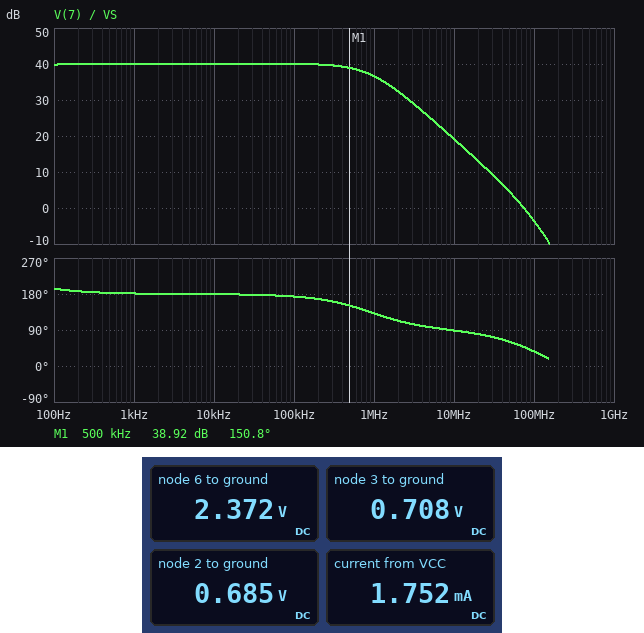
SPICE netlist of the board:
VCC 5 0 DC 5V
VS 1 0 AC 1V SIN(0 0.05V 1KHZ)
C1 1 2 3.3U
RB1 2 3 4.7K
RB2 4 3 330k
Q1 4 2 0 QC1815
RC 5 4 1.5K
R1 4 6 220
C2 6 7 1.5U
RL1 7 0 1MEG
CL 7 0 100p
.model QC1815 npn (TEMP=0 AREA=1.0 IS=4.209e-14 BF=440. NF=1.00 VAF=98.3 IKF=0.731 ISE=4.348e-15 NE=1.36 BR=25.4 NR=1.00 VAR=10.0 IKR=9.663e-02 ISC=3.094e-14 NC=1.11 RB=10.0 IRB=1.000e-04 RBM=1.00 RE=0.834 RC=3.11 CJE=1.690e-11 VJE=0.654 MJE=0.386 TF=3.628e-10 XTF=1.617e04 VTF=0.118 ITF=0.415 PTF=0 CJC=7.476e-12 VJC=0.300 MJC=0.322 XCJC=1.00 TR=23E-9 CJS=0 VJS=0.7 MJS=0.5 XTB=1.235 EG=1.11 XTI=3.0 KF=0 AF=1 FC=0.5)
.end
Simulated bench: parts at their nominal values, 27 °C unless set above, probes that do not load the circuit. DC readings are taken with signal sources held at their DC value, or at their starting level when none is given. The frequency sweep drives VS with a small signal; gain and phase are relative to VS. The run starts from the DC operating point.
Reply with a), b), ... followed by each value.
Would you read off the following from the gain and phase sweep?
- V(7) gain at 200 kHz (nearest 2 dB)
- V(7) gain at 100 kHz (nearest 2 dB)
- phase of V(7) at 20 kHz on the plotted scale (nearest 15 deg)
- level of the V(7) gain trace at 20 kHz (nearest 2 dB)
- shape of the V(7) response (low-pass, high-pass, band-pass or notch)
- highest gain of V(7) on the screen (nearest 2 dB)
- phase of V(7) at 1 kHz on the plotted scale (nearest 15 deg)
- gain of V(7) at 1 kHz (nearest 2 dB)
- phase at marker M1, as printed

a) 40 dB
b) 40 dB
c) 180 deg
d) 40 dB
e) low-pass
f) 40 dB
g) 180 deg
h) 40 dB
i) 150.8 deg
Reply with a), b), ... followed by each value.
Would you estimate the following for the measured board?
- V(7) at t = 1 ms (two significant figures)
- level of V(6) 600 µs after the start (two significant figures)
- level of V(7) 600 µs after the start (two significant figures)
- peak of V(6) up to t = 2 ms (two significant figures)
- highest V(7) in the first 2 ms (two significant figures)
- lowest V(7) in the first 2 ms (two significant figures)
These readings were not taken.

a) 1.5 V
b) 4.7 V
c) 2.3 V
d) 4.9 V
e) 2.5 V
f) -2.3 V
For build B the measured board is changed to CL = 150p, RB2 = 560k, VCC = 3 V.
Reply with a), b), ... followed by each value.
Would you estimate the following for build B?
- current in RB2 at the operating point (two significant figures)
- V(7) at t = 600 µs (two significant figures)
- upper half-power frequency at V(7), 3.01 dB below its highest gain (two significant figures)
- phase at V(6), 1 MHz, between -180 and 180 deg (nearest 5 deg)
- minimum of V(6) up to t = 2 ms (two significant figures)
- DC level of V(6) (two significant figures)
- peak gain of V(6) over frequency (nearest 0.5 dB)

a) 2.2 µA
b) 910 mV
c) 610 kHz
d) 120 deg
e) 28 mV
f) 1.9 V
g) 33.0 dB
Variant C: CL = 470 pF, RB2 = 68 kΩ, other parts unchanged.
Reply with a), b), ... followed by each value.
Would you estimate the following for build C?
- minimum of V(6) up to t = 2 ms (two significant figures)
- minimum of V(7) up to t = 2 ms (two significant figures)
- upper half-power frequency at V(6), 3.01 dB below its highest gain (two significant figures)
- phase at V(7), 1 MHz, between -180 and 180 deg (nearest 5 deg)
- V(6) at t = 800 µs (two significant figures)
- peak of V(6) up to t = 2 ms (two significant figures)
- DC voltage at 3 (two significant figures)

a) 31 mV
b) -1.2 V
c) 200 kHz
d) 100 deg
e) 4.7 V
f) 4.8 V
g) 730 mV
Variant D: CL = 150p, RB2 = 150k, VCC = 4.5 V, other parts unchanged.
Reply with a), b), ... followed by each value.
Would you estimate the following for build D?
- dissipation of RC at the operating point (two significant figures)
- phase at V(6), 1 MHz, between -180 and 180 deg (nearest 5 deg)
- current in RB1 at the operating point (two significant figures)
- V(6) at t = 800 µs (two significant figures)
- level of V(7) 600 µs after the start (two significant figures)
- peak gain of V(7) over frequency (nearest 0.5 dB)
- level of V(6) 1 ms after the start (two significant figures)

a) 5.7 mW
b) 120 deg
c) 5.7 µA
d) 4.3 V
e) 2.6 V
f) 41.0 dB
g) 3.3 V
